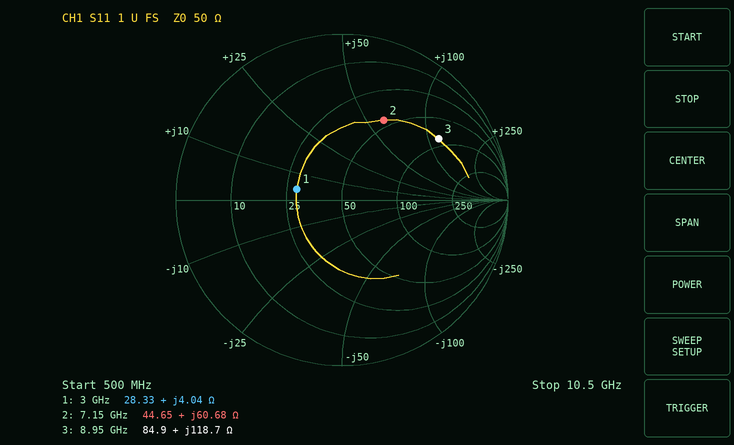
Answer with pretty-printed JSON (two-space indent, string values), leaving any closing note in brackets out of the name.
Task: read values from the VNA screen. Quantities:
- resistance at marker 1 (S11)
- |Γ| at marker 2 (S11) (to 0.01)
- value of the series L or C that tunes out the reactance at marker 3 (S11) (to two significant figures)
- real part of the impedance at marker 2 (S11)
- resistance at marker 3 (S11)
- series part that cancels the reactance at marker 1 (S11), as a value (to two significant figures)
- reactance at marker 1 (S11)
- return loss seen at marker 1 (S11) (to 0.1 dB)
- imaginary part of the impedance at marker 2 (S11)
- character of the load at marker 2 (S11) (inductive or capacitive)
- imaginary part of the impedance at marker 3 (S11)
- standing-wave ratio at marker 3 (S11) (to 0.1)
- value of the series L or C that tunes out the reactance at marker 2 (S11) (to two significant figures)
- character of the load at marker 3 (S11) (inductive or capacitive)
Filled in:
{
  "resistance at marker 1": "28.33 Ω",
  "|Γ| at marker 2 (S11)": "0.54",
  "value of the series L or C that tunes out the reactance at marker 3 (S11)": "150 fF",
  "real part of the impedance at marker 2": "44.65 Ω",
  "resistance at marker 3": "84.9 Ω",
  "series part that cancels the reactance at marker 1 (S11), as a value": "13 pF",
  "reactance at marker 1": "+4.04 Ω",
  "return loss seen at marker 1 (S11)": "11.0 dB",
  "imaginary part of the impedance at marker 2": "+60.68 Ω",
  "character of the load at marker 2 (S11)": "inductive",
  "imaginary part of the impedance at marker 3": "+118.7 Ω",
  "standing-wave ratio at marker 3 (S11)": "5.4",
  "value of the series L or C that tunes out the reactance at marker 2 (S11)": "370 fF",
  "character of the load at marker 3 (S11)": "inductive"
}
